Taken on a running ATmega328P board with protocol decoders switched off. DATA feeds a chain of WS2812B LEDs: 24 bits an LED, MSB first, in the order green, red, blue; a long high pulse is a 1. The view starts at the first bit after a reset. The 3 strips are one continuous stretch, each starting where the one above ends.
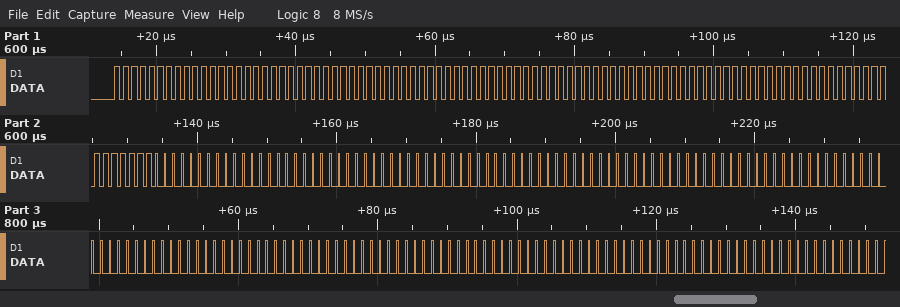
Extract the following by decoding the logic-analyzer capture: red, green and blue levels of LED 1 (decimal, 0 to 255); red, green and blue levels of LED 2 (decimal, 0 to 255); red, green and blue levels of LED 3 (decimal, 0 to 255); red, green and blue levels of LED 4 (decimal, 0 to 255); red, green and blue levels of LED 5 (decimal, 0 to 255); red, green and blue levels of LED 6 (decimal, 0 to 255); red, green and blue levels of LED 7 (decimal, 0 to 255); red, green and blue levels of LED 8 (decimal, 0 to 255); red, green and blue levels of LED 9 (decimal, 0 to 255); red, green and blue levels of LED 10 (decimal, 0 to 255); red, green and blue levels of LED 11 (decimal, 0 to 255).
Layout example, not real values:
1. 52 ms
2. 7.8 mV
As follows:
1. 255, 255, 255
2. 255, 255, 255
3. 255, 255, 255
4. 255, 255, 255
5. 0, 0, 0
6. 0, 0, 0
7. 0, 0, 0
8. 0, 0, 0
9. 0, 0, 0
10. 0, 0, 0
11. 0, 0, 0
